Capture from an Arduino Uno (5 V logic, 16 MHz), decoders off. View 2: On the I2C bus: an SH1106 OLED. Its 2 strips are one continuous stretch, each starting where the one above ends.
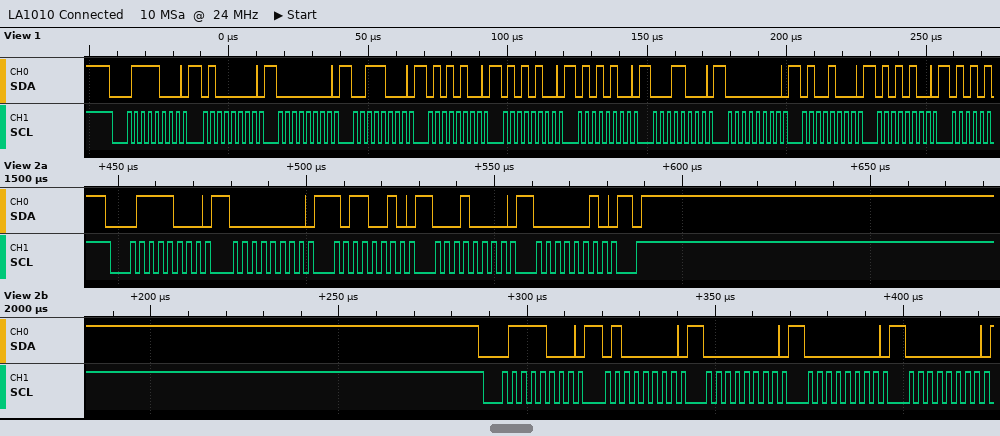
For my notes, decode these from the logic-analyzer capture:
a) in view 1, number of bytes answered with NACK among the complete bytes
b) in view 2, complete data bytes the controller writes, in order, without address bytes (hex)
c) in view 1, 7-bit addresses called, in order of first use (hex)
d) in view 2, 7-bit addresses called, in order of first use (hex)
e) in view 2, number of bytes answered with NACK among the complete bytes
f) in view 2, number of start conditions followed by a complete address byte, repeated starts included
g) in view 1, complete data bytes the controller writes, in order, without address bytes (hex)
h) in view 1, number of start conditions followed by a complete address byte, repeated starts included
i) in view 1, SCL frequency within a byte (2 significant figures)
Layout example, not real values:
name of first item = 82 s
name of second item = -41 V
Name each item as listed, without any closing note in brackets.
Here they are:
in view 1, number of bytes answered with NACK among the complete bytes = 0
in view 2, complete data bytes the controller writes, in order, without address bytes = 00 B2 10 02 40 00 00 00
in view 1, 7-bit addresses called, in order of first use = 0x3C
in view 2, 7-bit addresses called, in order of first use = 0x3C
in view 2, number of bytes answered with NACK among the complete bytes = 0
in view 2, number of start conditions followed by a complete address byte, repeated starts included = 2
in view 1, complete data bytes the controller writes, in order, without address bytes = 40 00 38 54 54 54 18 00 48 54
in view 1, number of start conditions followed by a complete address byte, repeated starts included = 1
in view 1, SCL frequency within a byte = 400 kHz
